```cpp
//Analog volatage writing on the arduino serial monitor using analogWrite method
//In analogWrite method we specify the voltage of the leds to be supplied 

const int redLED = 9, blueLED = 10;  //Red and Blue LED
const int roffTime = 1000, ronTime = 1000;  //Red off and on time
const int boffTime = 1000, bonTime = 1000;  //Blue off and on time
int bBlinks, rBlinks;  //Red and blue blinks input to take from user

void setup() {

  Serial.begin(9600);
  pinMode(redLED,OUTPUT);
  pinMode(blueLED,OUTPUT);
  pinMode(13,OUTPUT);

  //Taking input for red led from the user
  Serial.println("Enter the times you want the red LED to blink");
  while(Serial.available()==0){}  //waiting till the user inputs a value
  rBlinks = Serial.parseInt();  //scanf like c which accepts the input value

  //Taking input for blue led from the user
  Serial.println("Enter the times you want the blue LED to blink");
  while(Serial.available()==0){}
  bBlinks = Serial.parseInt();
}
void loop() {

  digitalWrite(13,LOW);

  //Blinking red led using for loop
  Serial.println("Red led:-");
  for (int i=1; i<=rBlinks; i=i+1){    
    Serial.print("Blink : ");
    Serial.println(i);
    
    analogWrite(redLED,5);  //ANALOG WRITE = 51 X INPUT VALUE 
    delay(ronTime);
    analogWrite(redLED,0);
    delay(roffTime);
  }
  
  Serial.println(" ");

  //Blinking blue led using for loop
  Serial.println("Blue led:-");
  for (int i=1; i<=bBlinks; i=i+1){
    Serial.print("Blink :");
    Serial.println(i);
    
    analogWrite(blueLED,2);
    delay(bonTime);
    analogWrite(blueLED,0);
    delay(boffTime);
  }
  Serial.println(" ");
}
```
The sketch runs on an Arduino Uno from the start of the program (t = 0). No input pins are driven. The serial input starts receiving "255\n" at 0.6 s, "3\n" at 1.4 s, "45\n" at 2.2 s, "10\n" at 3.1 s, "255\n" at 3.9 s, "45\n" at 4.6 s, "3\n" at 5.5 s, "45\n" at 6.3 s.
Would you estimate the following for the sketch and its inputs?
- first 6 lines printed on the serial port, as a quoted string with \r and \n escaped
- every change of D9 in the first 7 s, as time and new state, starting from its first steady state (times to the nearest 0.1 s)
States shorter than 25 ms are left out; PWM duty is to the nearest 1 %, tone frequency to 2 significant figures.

"Enter the times you want the red LED to blink\r\nEnter the times you want the blue LED to blink\r\nRed led:-\r\nBlink : 1\r\nBlink : 2\r\nBlink : 3\r\n"
0 s low; 1.4 s PWM 2 %; 2.4 s low; 3.4 s PWM 2 %; 4.4 s low; 5.4 s PWM 2 %; 6.4 s low
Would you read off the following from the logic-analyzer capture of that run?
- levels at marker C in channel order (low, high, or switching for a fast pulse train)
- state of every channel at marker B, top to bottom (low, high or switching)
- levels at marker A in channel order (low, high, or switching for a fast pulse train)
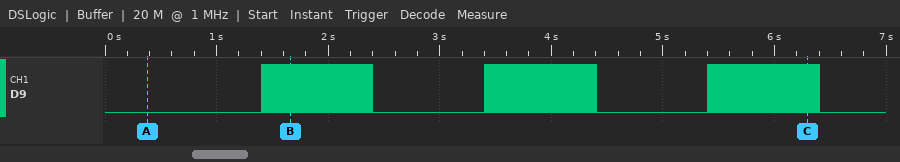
D9 switching
D9 switching
D9 low
